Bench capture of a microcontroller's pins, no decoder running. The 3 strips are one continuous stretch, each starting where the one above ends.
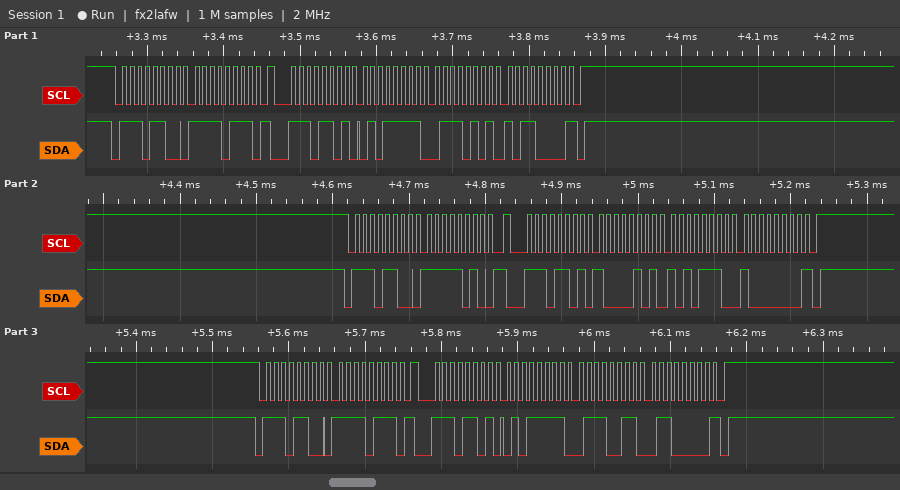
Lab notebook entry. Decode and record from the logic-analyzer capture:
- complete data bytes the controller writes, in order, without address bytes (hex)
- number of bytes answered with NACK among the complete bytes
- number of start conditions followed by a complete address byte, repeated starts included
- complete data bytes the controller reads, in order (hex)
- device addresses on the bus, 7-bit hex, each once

F7 FA F7
3
6
5F 75 B0 85 AE 80 5F 73 60
0x76
